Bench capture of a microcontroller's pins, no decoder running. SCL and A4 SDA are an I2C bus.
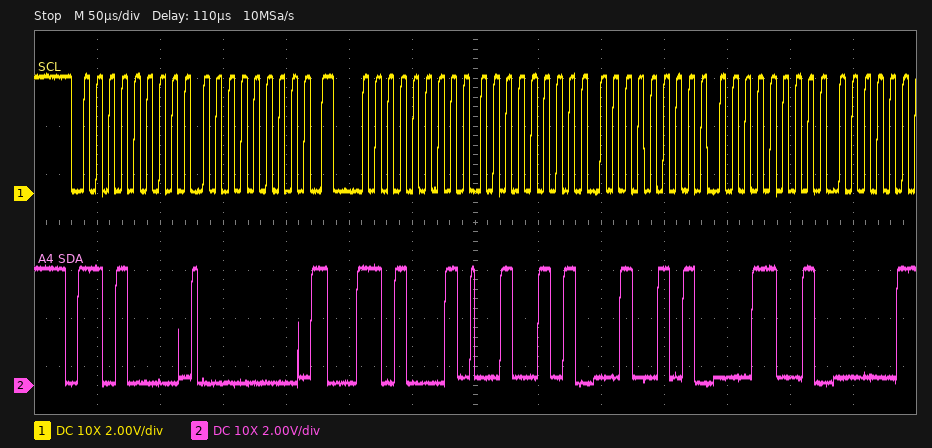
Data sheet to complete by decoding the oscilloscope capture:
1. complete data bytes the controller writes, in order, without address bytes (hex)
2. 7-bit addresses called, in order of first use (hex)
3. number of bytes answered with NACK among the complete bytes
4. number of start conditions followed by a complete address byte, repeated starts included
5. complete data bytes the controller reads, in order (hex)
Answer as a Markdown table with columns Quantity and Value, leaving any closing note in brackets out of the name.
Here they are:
| Quantity | Value |
|---|---|
| complete data bytes the controller writes, in order, without address bytes | 00 |
| 7-bit addresses called, in order of first use | 0x68 |
| number of bytes answered with NACK among the complete bytes | 0 |
| number of start conditions followed by a complete address byte, repeated starts included | 2 |
| complete data bytes the controller reads, in order | 25 25 19 |
